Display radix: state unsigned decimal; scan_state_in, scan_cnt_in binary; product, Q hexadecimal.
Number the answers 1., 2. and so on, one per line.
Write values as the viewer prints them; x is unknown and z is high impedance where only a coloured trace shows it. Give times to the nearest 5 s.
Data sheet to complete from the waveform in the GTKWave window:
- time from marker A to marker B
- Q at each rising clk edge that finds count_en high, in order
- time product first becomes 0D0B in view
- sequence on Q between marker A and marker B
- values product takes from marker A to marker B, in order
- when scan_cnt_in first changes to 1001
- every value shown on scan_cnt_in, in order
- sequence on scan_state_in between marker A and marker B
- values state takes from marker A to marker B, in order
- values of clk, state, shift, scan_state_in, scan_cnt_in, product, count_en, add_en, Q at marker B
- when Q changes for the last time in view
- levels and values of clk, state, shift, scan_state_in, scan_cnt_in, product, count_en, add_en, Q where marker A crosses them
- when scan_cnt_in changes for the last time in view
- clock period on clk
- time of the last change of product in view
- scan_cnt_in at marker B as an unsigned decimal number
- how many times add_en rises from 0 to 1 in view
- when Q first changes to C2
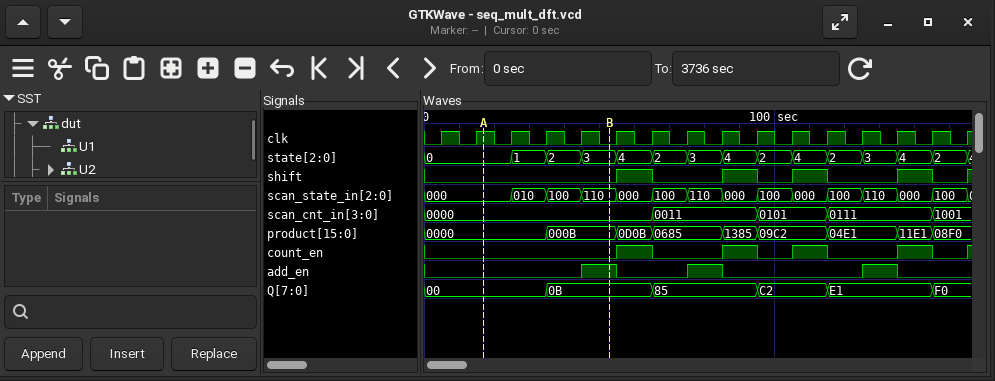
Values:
1. 35 s
2. 0B, 85, C2, E1
3. 55 s
4. 00, 0B
5. 0000, 000B
6. 145 s
7. 0000, 0011, 0101, 0111, 1001
8. 000, 010, 100, 110
9. 0, 1, 2, 3
10. clk=0, state=3, shift=0, scan_state_in=110, scan_cnt_in=0000, product=000B, count_en=0, add_en=1, Q=0B
11. 145 s
12. clk=1, state=0, shift=0, scan_state_in=000, scan_cnt_in=0000, product=0000, count_en=0, add_en=0, Q=00
13. 145 s
14. 10 s
15. 145 s
16. 0
17. 3
18. 95 s
